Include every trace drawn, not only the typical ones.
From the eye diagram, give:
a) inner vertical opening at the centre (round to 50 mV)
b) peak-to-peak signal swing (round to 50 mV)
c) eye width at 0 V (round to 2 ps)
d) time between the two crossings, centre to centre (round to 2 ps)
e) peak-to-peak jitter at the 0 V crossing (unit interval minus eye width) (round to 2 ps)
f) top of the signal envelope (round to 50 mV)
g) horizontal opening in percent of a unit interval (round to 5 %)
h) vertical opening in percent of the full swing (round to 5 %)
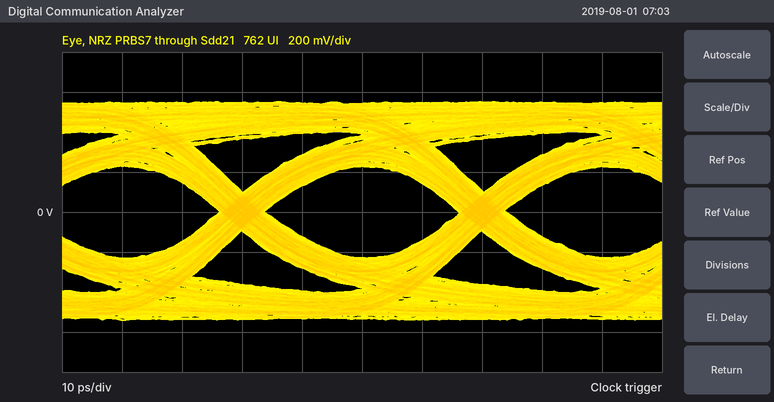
450 mV
1.10 V
32 ps
40 ps
8 ps
550 mV
80 %
40 %
